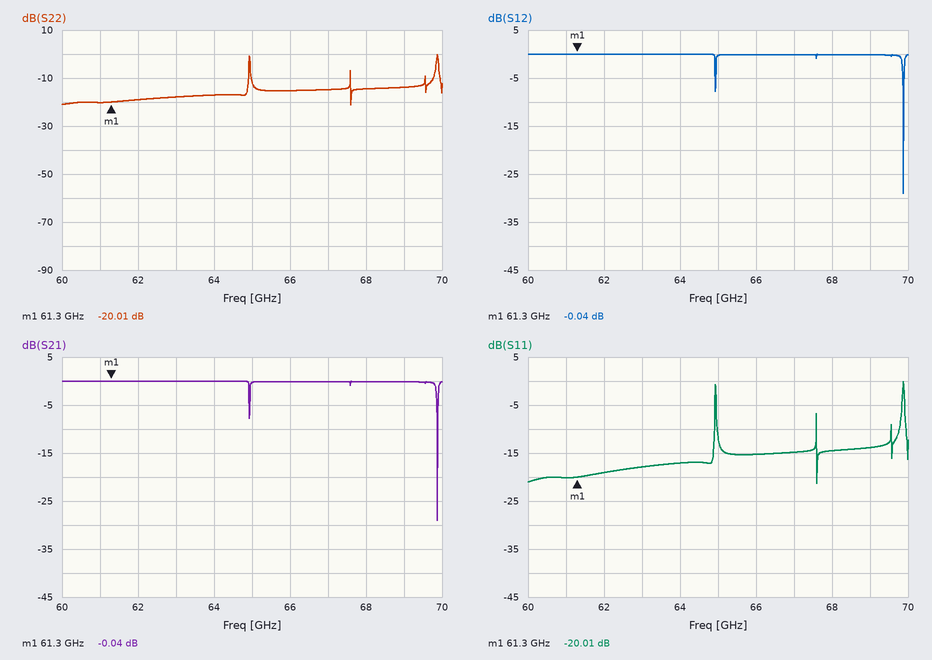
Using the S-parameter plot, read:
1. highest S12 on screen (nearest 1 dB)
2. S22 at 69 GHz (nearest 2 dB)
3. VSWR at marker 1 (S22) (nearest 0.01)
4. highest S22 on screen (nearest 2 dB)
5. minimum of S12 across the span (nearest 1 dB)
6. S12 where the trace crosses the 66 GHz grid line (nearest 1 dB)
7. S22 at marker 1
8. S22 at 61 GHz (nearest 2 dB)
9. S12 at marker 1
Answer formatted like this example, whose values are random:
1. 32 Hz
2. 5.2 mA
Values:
1. 0 dB
2. -14 dB
3. 1.22
4. 0 dB
5. -29 dB
6. 0 dB
7. -20.01 dB
8. -20 dB
9. -0.04 dB
